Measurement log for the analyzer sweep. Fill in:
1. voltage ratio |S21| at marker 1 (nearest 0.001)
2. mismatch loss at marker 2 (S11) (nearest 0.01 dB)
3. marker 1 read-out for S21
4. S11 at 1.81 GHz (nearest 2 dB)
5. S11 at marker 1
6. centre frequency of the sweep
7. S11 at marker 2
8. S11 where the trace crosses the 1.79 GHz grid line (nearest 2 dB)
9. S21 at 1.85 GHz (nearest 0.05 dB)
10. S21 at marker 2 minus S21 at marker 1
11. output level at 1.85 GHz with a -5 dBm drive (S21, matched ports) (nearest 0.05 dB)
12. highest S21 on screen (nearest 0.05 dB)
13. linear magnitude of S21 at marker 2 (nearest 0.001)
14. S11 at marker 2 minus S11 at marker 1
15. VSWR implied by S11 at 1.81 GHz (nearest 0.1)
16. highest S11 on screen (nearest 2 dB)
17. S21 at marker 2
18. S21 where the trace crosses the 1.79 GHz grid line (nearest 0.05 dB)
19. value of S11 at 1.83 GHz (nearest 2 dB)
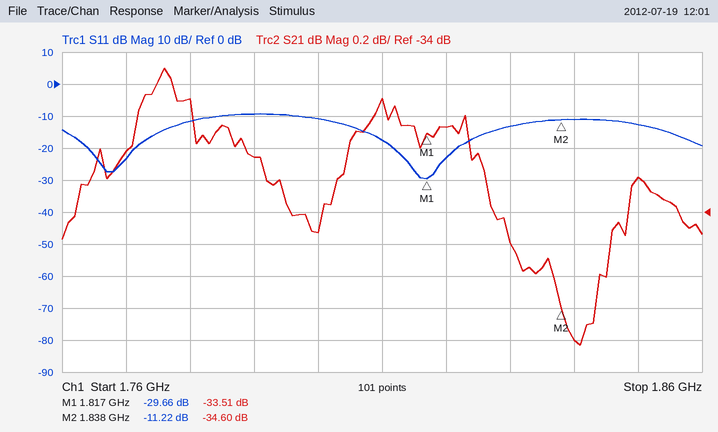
0.021
0.34 dB
-33.51 dB
-18 dB
-29.66 dB
1.81 GHz
-11.22 dB
-10 dB
-33.80 dB
-1.09 dB
-38.80 dBm
-33.10 dB
0.019
18.44 dB
1.3
-10 dB
-34.60 dB
-33.65 dB
-14 dB
